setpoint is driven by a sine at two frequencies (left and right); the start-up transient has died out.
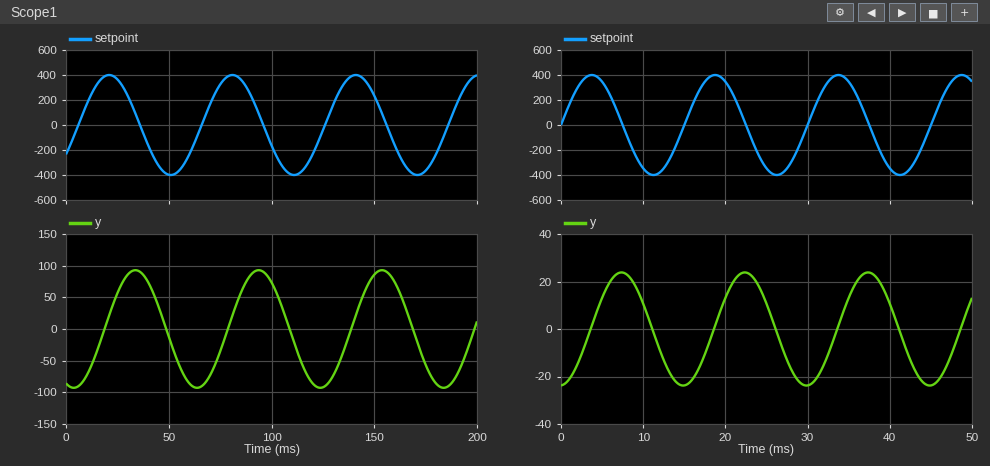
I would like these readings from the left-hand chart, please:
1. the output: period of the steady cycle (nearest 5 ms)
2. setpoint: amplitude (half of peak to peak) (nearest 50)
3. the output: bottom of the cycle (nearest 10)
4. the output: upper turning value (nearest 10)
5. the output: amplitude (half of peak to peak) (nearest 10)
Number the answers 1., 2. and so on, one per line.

1. 60 ms
2. 400
3. -90
4. 90
5. 90
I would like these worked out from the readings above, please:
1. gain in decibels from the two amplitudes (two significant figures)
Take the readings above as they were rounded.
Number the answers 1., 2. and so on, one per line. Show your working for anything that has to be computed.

1. 20 log10(90 / 400) = -13 dB
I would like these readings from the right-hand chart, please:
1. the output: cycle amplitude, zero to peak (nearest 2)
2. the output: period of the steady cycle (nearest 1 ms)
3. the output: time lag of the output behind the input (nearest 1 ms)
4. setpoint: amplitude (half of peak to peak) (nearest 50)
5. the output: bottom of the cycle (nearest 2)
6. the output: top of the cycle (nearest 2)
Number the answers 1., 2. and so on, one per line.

1. 24
2. 15 ms
3. 4 ms
4. 400
5. -24
6. 24
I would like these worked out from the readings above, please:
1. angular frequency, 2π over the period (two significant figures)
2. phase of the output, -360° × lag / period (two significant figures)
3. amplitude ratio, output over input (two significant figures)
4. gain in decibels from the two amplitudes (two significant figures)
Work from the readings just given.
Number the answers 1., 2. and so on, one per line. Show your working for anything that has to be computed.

1. 2π / 15 = 0.42 rad/ms
2. -360 × 4 / 15 = -96°
3. 24 / 400 = 0.060
4. 20 log10(24 / 400) = -24 dB
